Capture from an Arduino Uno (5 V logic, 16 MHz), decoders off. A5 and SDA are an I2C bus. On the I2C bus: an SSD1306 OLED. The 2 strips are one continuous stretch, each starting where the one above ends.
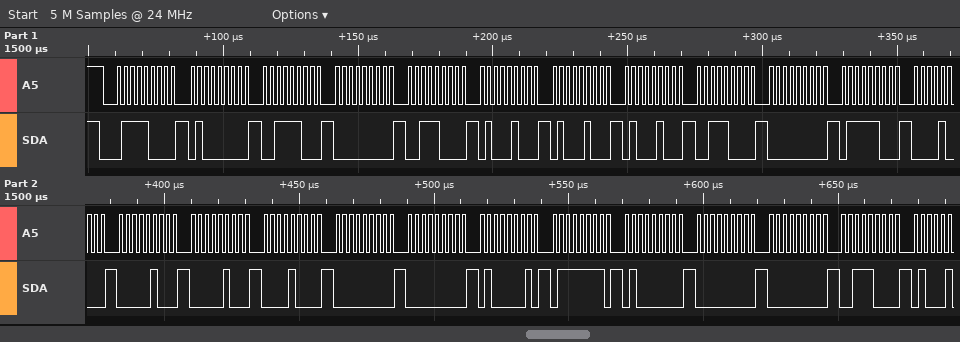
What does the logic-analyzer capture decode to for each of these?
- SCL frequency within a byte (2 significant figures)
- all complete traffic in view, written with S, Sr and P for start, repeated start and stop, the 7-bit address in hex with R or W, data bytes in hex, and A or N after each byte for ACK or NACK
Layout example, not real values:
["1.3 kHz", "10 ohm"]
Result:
["400 kHz", "S 3CW A 40 A 3C A 00 A 38 A 44 A 44 A 44 A 38 A 00 A 7C A 08 A 04 A 04 A 08 A 00 A 00 A 41 A 7F A 40 A 00 A 00 A 38 A"]
